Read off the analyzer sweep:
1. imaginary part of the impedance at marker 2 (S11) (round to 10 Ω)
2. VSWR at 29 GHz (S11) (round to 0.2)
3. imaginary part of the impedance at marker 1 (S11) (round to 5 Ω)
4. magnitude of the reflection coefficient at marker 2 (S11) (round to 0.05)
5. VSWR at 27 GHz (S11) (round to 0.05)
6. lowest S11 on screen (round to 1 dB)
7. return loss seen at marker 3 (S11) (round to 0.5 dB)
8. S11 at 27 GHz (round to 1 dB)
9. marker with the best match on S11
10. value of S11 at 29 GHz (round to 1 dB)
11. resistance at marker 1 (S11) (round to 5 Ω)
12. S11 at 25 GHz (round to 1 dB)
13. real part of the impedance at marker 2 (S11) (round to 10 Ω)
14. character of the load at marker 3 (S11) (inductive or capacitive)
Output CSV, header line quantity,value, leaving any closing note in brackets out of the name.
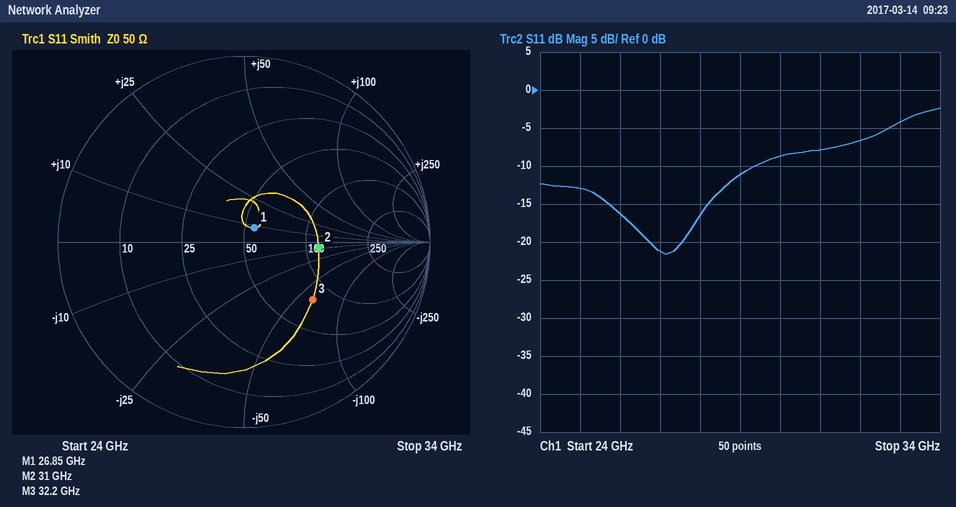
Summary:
quantity,value
imaginary part of the impedance at marker 2 (S11),-10 Ω
VSWR at 29 GHz (S11),1.8
imaginary part of the impedance at marker 1 (S11),+10 Ω
magnitude of the reflection coefficient at marker 2 (S11),0.40
VSWR at 27 GHz (S11),1.20
lowest S11 on screen,-22 dB
return loss seen at marker 3 (S11),6.5 dB
S11 at 27 GHz,-21 dB
marker with the best match on S11,marker 1
value of S11 at 29 GHz,-11 dB
resistance at marker 1 (S11),55 Ω
S11 at 25 GHz,-13 dB
real part of the impedance at marker 2 (S11),120 Ω
character of the load at marker 3 (S11),capacitive
